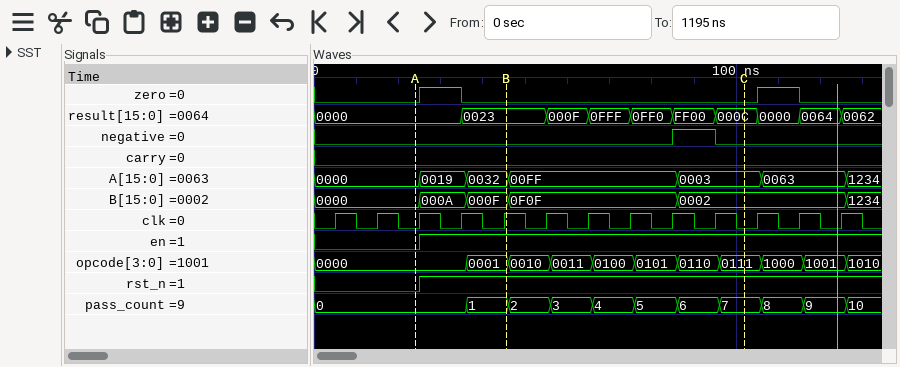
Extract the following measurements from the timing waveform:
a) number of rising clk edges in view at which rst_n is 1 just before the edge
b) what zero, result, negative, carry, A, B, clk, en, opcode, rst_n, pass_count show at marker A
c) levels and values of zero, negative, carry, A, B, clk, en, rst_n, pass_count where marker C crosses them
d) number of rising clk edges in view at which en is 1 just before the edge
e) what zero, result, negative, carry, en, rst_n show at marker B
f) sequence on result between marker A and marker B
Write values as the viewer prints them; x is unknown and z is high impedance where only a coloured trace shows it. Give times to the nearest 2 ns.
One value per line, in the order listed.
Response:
10
zero=0, result=0000, negative=0, carry=0, A=0000, B=0000, clk=0, en=0, opcode=0000, rst_n=0, pass_count=0
zero=0, negative=0, carry=0, A=0003, B=0002, clk=0, en=1, rst_n=1, pass_count=7
10
zero=0, result=0023, negative=0, carry=0, en=1, rst_n=1
0000, 0023
